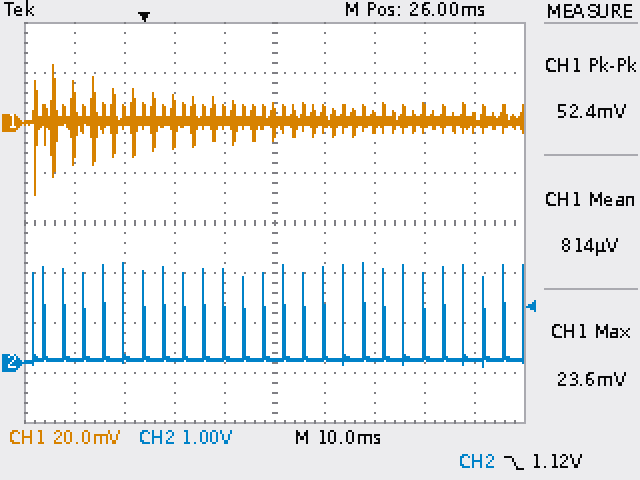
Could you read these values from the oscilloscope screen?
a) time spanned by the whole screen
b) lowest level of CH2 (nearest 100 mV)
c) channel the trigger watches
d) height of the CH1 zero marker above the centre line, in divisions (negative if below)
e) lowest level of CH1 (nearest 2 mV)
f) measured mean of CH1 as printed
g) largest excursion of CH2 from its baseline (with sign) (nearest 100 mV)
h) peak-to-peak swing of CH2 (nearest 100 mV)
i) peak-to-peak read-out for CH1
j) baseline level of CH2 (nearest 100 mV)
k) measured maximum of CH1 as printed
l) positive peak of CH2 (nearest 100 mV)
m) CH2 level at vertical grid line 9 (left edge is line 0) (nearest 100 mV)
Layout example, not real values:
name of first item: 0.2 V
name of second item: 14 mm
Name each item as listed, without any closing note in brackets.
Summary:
time spanned by the whole screen: 100 ms
lowest level of CH2: -100 mV
channel the trigger watches: CH2
height of the CH1 zero marker above the centre line, in divisions: +2.0 div
lowest level of CH1: -28 mV
measured mean of CH1 as printed: 814 µV
largest excursion of CH2 from its baseline (with sign): +1.9 V
peak-to-peak swing of CH2: 2.1 V
peak-to-peak read-out for CH1: 52.4 mV
baseline level of CH2: 100 mV
measured maximum of CH1 as printed: 23.6 mV
positive peak of CH2: 2.0 V
CH2 level at vertical grid line 9 (left edge is line 0): 100 mV
